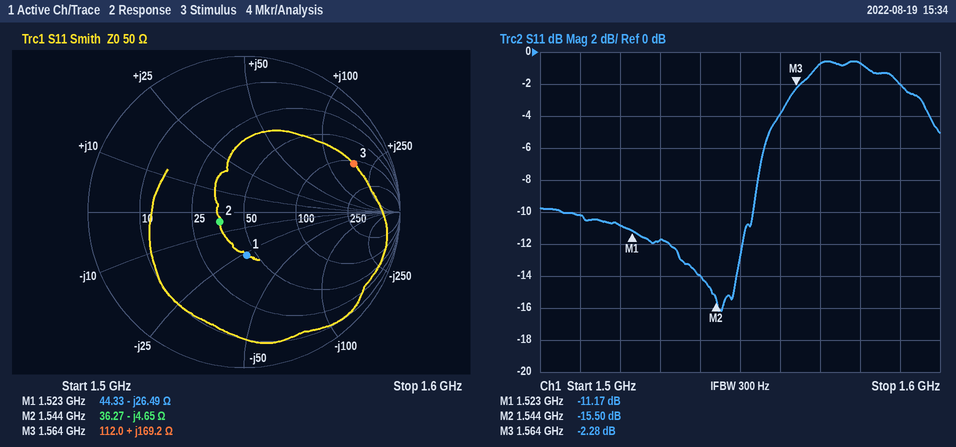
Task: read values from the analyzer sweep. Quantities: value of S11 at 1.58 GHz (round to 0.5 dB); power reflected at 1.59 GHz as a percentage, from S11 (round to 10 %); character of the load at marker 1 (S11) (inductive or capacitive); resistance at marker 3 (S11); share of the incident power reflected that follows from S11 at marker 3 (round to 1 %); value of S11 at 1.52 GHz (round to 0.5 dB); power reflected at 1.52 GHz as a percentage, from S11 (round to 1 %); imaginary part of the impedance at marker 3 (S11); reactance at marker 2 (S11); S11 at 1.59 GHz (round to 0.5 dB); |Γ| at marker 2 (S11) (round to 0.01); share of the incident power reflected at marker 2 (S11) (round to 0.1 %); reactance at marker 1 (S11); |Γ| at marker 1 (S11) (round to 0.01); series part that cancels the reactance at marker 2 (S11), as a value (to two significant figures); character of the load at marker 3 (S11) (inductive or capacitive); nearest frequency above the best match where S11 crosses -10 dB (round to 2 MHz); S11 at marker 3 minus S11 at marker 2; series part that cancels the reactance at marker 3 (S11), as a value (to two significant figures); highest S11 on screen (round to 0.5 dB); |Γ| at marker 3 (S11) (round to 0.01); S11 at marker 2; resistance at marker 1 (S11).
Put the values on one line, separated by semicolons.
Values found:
-0.5 dB; 60 %; capacitive; 112.0 Ω; 59 %; -11.0 dB; 8 %; +169.2 Ω; -4.65 Ω; -2.0 dB; 0.17; 2.8 %; -26.49 Ω; 0.28; 480 pH; inductive; 1.554 GHz; 13.22 dB; 600 fF; -0.5 dB; 0.77; -15.50 dB; 44.33 Ω
